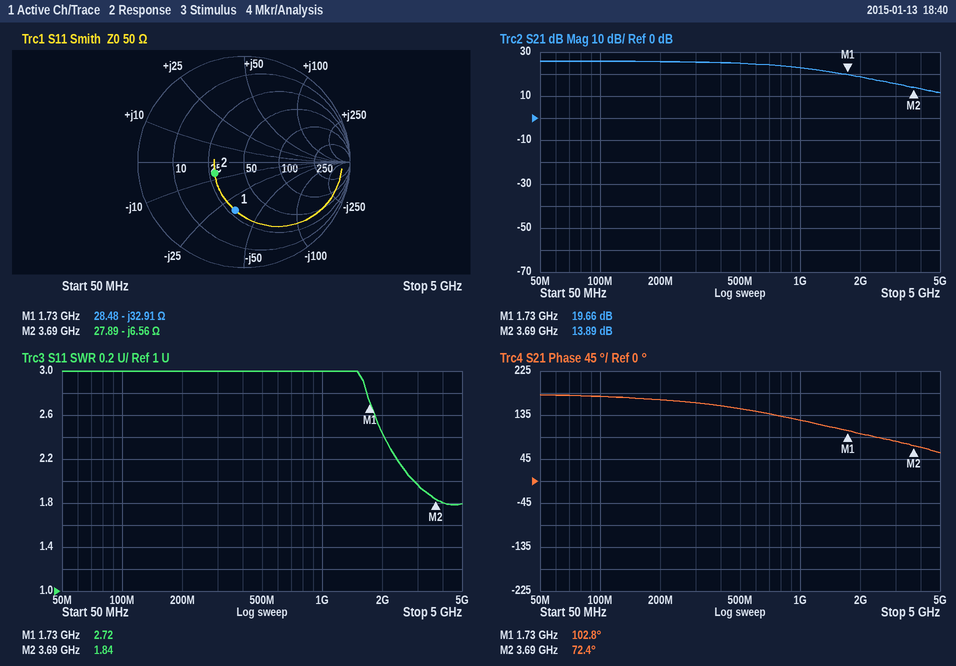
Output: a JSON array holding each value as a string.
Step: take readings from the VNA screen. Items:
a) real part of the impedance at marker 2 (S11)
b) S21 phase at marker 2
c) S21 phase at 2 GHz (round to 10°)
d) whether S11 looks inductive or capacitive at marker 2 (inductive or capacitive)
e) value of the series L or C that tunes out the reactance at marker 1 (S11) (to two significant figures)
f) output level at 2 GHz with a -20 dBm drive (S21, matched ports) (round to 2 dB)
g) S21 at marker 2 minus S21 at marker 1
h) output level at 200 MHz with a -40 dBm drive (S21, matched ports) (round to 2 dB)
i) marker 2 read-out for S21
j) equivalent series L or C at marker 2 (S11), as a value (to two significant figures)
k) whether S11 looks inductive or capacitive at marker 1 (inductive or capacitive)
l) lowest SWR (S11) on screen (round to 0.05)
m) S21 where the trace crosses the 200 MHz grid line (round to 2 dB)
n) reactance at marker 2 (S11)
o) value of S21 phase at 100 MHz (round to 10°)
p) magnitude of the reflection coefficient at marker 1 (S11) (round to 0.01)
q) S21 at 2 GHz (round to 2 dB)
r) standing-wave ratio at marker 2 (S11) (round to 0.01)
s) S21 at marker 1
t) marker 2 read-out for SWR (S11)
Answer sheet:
["27.89 Ω", "72.4°", "100°", "capacitive", "3.0 nH", "-2 dBm", "-5.77 dB", "-14 dBm", "13.89 dB", "6.6 pF", "capacitive", "1.80", "26 dB", "-6.56 Ω", "170°", "0.46", "18 dB", "1.84", "19.66 dB", "1.84"]
